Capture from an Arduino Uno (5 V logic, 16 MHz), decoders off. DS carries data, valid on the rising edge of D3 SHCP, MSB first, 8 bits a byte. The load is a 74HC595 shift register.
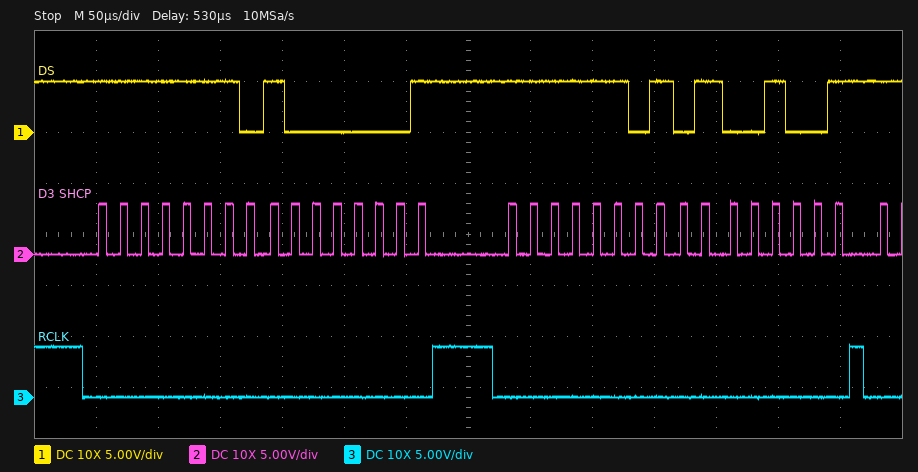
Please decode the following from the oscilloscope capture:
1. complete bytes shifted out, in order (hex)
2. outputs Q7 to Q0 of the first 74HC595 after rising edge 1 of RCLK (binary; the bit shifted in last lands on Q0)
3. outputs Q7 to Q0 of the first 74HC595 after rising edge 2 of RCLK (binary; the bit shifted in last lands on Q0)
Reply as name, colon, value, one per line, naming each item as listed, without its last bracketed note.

complete bytes shifted out, in order: FE 81 FD 49
outputs Q7 to Q0 of the first 74HC595 after rising edge 1 of RCLK: 10000001
outputs Q7 to Q0 of the first 74HC595 after rising edge 2 of RCLK: 01001001
